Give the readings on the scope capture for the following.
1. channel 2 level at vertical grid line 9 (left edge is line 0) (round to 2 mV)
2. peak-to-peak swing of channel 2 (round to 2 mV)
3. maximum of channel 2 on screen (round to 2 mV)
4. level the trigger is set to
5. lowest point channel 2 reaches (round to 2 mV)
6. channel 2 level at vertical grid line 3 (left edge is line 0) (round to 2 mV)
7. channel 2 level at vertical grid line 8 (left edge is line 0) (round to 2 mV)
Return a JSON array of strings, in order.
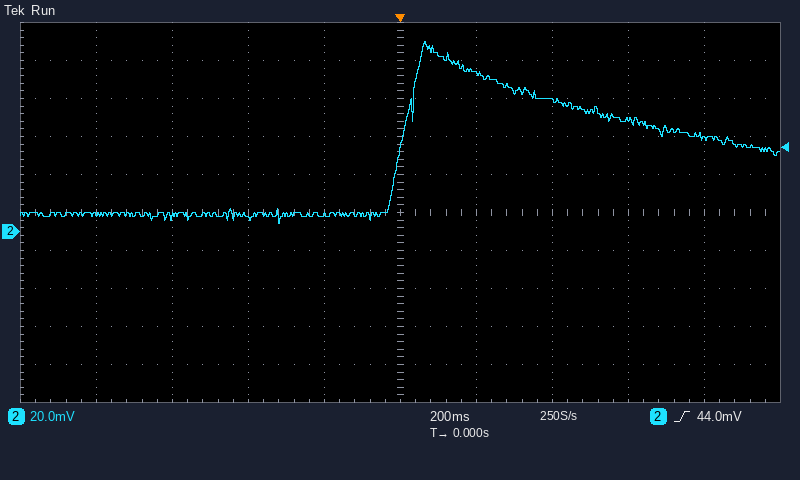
["50 mV", "96 mV", "100 mV", "44.0 mV", "4 mV", "8 mV", "58 mV"]
